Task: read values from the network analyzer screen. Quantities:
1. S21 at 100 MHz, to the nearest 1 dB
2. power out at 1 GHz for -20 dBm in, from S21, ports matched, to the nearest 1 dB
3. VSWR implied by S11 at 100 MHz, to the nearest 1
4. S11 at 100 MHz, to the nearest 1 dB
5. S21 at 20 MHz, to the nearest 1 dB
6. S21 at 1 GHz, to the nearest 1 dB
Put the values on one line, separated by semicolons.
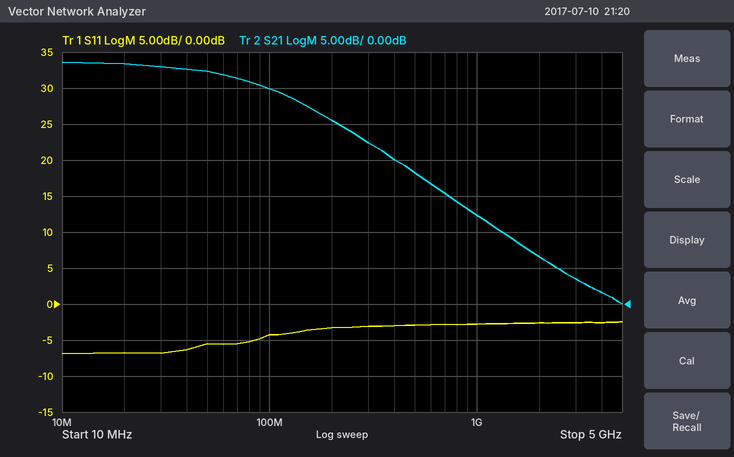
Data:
30 dB; -8 dBm; 4; -4 dB; 33 dB; 12 dB
